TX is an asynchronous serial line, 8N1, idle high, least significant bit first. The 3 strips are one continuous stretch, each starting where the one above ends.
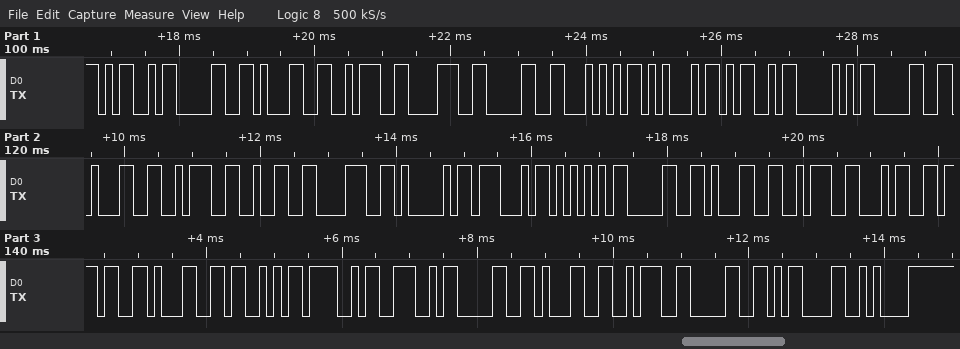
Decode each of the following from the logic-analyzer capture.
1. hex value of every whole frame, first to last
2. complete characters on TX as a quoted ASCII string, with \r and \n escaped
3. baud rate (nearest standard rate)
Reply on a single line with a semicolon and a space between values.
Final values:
4D 30 31 3A 38 30 54 45 4D 50 30 31 3A 32 38 41 47 55 30 31 3A 34 37 31 53 4F 4E 30 31 3A 30 0D 0A; "M01:80TEMP01:28AGU01:471SON01:0\r\n"; 9600 baud
